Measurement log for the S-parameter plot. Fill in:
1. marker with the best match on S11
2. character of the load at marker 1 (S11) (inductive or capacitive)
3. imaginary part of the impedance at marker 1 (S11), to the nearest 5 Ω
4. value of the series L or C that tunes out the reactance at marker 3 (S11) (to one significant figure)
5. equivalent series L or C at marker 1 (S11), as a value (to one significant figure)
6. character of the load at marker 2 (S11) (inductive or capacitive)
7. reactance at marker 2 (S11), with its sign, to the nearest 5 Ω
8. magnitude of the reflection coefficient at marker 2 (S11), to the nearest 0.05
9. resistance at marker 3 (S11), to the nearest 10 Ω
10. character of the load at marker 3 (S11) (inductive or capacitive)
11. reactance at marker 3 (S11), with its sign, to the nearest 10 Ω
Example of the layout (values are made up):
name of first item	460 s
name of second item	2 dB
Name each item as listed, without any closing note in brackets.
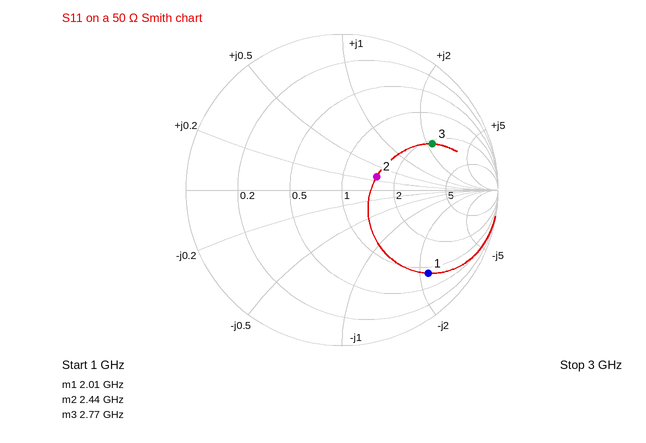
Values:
marker with the best match on S11	marker 2
character of the load at marker 1 (S11)	capacitive
imaginary part of the impedance at marker 1 (S11), to the nearest 5 Ω	-110 Ω
value of the series L or C that tunes out the reactance at marker 3 (S11)	500 fF
equivalent series L or C at marker 1 (S11), as a value	700 fF
character of the load at marker 2 (S11)	inductive
reactance at marker 2 (S11), with its sign, to the nearest 5 Ω	+15 Ω
magnitude of the reflection coefficient at marker 2 (S11), to the nearest 0.05	0.25
resistance at marker 3 (S11), to the nearest 10 Ω	110 Ω
character of the load at marker 3 (S11)	inductive
reactance at marker 3 (S11), with its sign, to the nearest 10 Ω	+110 Ω
